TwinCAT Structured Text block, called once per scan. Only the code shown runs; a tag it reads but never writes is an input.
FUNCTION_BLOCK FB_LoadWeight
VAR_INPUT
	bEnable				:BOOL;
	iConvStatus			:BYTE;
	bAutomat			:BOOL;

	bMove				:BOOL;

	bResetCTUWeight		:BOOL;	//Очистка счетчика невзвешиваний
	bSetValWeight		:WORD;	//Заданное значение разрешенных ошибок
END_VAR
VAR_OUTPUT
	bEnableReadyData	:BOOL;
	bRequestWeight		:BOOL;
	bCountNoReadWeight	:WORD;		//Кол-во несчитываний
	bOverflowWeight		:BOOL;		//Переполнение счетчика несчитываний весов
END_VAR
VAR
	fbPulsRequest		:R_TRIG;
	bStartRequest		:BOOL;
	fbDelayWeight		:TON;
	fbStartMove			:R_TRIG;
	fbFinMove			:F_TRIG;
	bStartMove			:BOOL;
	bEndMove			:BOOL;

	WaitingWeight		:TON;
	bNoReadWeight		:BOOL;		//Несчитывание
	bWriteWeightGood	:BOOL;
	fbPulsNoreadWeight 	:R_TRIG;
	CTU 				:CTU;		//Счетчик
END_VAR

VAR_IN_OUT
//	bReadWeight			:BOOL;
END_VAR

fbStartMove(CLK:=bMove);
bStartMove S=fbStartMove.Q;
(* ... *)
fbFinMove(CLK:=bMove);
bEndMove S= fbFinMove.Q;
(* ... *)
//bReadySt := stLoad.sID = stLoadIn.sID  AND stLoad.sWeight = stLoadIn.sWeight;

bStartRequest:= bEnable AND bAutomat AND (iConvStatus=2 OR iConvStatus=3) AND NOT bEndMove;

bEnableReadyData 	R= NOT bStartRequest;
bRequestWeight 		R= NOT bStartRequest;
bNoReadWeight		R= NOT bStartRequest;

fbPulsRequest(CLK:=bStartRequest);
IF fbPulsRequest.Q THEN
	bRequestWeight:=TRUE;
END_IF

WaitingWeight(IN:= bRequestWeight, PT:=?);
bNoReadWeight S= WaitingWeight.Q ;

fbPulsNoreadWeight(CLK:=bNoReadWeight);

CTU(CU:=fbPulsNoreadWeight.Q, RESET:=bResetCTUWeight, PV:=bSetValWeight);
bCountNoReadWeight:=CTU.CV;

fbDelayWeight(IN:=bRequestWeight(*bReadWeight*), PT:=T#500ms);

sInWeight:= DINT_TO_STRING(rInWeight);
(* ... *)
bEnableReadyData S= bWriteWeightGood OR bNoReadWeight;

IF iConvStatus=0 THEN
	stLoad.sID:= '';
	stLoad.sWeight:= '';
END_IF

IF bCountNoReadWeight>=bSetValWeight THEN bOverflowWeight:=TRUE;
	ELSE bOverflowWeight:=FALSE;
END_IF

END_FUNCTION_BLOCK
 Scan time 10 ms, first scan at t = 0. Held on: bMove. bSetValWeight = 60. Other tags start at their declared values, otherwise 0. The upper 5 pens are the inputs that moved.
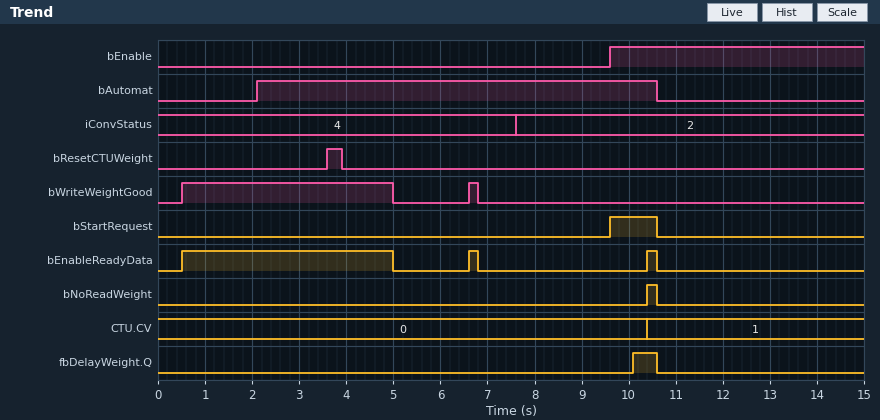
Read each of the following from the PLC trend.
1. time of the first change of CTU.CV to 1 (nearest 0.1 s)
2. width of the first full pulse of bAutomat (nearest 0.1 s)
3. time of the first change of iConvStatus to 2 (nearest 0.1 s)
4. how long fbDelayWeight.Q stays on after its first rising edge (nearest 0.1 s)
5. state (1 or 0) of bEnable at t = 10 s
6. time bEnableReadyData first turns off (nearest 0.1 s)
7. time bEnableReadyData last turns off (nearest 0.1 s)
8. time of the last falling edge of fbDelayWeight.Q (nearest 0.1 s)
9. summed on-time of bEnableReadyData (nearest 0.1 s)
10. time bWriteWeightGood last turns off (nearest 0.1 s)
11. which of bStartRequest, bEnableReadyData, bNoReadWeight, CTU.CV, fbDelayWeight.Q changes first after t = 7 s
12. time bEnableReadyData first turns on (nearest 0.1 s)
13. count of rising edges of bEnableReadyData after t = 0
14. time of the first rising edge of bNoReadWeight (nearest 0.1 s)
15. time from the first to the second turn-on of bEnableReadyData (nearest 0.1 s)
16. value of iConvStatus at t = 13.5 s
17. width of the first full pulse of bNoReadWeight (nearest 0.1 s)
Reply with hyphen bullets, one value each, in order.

- 10.4 s
- 8.5 s
- 7.6 s
- 0.5 s
- 1
- 5.0 s
- 10.6 s
- 10.6 s
- 4.9 s
- 6.8 s
- bStartRequest
- 0.5 s
- 3
- 10.4 s
- 6.1 s
- 2
- 0.2 s
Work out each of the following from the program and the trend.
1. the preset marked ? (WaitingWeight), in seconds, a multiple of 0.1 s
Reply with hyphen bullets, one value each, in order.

- 0.8 s
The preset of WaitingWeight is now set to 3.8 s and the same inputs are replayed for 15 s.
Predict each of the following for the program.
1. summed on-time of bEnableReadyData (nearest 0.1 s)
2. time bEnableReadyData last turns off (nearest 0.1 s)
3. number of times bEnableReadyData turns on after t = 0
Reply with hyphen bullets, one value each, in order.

- 4.7 s
- 6.8 s
- 2
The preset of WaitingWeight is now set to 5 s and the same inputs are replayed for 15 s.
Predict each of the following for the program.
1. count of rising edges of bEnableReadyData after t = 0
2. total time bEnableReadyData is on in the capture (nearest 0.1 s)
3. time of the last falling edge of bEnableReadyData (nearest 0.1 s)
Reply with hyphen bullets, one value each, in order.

- 2
- 4.7 s
- 6.8 s
